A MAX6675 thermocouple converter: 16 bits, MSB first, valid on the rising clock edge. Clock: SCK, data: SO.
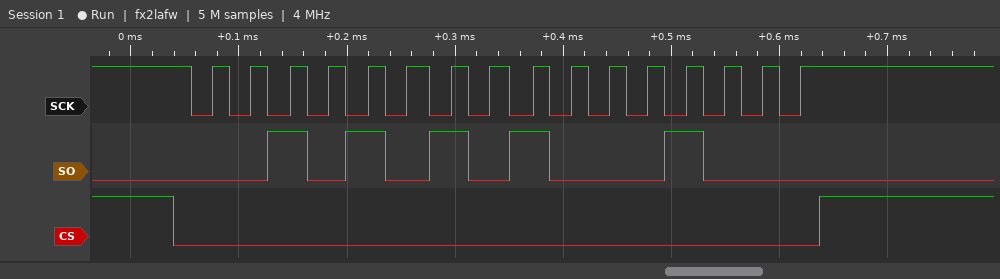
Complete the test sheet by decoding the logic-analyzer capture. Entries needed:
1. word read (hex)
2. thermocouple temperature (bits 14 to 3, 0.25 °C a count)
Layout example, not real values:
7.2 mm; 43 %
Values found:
0x2A88; 340.25 °C
